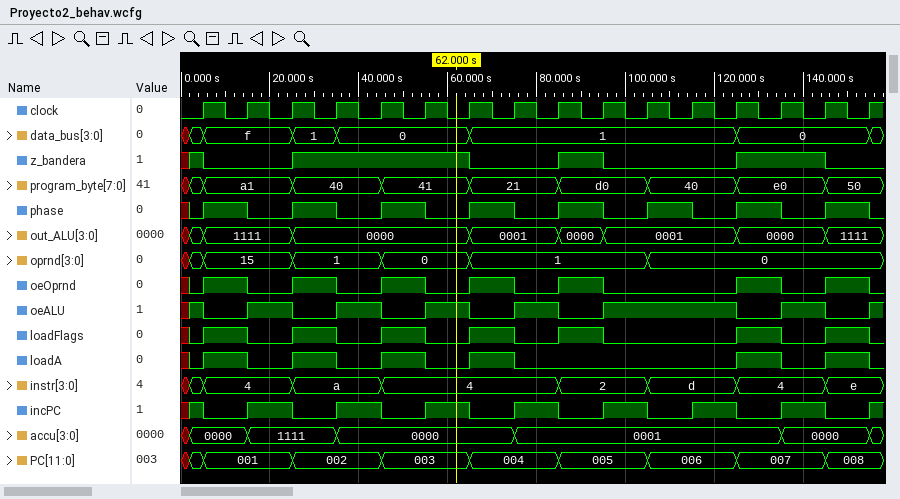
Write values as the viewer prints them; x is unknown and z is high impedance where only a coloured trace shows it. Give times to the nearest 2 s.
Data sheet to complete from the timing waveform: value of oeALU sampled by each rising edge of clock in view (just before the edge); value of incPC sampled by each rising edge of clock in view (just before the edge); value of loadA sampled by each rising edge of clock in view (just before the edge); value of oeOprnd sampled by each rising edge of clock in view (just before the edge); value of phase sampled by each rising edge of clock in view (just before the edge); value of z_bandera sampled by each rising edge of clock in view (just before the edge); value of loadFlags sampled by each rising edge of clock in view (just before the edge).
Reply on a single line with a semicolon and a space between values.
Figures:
1 0 1 0 1 0 1 0 1 0 1 1 1 0 1 0; 1 0 1 0 1 0 1 0 1 0 1 0 1 0 1 0; 0 1 0 1 0 1 0 1 0 0 0 0 0 1 0 1; 0 1 0 1 0 1 0 1 0 1 0 0 0 1 0 1; 0 1 0 1 0 1 0 1 0 1 0 1 0 1 0 1; 1 0 0 1 1 1 1 0 0 1 0 0 0 1 1 0; 0 1 0 1 0 1 0 1 0 1 0 0 0 1 0 1
